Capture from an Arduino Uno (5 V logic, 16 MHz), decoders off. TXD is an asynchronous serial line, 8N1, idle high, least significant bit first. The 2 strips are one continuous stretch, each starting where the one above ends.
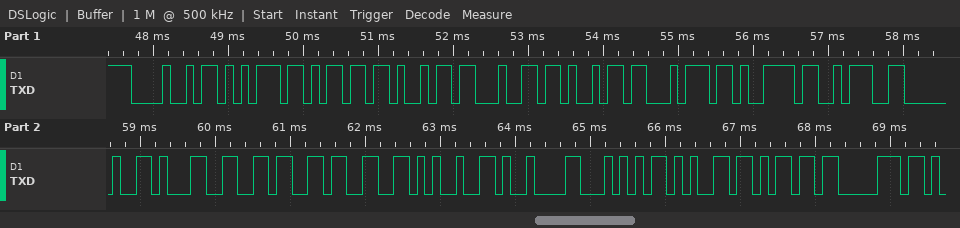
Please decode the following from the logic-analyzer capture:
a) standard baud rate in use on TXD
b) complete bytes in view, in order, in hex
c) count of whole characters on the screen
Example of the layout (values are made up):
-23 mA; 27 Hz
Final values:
9600 baud; 48 75 6D 69 64 69 74 79 3A 20 31 36 33 25 09 54 65 6D 70; 19
